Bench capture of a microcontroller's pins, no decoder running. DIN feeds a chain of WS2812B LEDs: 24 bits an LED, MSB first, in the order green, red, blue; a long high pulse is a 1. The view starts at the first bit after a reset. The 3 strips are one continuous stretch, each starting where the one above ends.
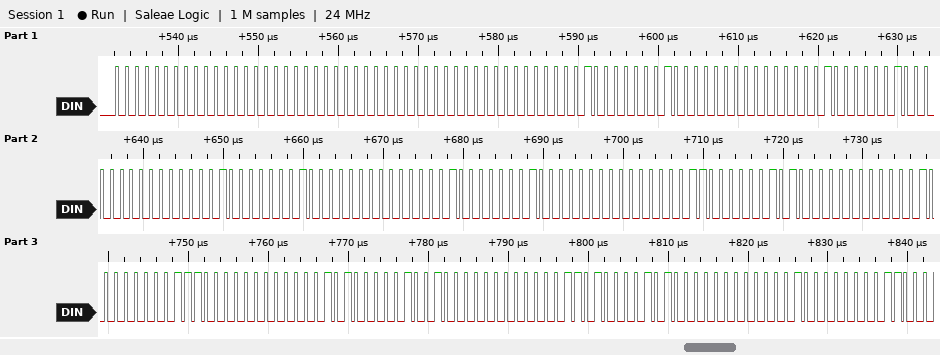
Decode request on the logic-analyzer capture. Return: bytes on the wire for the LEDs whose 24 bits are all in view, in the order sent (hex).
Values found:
00 00 00 00 00 01 01 00 01 02 00 02 02 00 04 04 00 06 05 00 08 07 00 0A 09 00 0D 0A 00 10
